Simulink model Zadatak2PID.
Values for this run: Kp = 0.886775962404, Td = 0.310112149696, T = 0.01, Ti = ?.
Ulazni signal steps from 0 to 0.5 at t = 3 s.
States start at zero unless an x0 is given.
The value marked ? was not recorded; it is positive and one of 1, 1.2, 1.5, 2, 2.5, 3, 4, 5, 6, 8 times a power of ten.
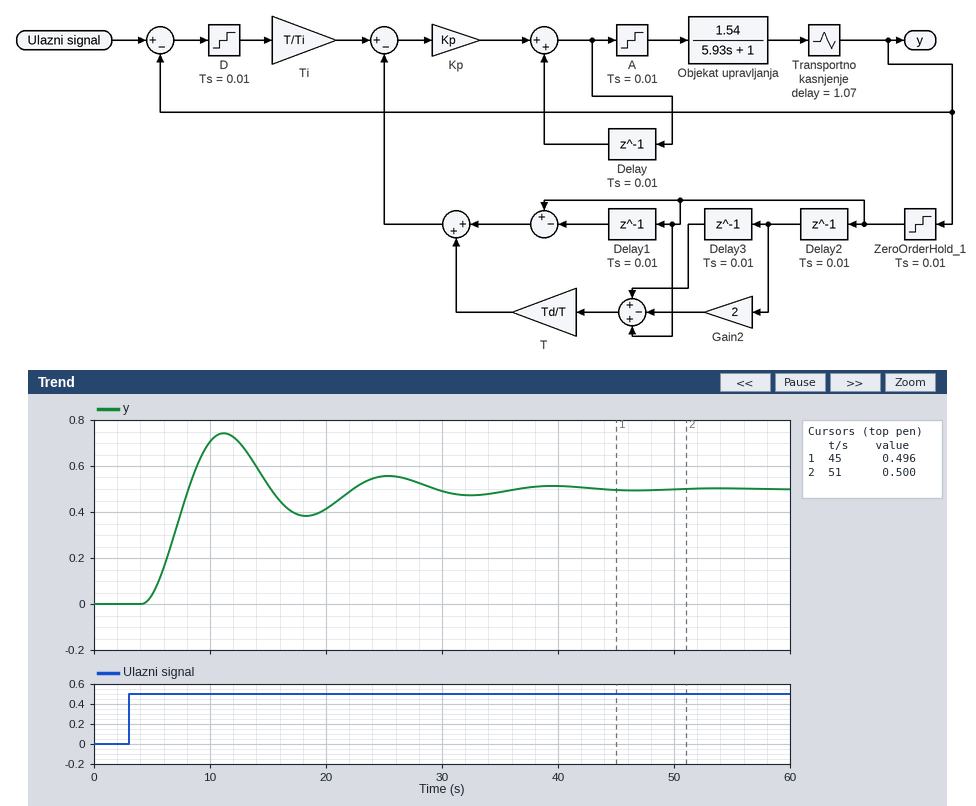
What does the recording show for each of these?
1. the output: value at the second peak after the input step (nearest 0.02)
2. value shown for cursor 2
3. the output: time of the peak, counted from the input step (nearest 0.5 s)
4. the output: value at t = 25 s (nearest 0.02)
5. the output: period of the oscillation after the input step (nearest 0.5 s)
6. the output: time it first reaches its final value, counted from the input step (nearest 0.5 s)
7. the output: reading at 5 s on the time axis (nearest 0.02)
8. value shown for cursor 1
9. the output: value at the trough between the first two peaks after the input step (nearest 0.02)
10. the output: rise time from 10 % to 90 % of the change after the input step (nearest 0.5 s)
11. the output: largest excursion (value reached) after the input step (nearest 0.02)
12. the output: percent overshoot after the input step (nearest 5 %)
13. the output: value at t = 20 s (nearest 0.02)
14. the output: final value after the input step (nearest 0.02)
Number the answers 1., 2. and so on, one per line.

1. 0.56
2. 0.500
3. 8.0 s
4. 0.56
5. 14.0 s
6. 5.0 s
7. 0.04
8. 0.496
9. 0.38
10. 2.5 s
11. 0.74
12. 50 %
13. 0.42
14. 0.50
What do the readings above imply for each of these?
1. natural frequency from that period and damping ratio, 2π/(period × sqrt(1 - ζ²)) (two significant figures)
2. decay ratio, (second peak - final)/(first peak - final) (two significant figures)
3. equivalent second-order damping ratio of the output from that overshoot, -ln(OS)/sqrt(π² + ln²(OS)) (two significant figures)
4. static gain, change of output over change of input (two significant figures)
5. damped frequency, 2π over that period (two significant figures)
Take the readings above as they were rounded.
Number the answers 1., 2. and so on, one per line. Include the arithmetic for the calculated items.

1. 2π / (14 × sqrt(1 - 0.22²)) = 0.46 rad/s
2. (0.56 - 0.5) / (0.74 - 0.5) = 0.25
3. ln(0.5) = -0.693; 0.693 / sqrt(9.870 + 0.480) = 0.22
4. (0.5 - 0) / (0.5 - 0) = 1.0
5. 2π / 14 = 0.45 rad/s
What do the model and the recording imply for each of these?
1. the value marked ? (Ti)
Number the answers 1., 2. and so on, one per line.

1. 1.2
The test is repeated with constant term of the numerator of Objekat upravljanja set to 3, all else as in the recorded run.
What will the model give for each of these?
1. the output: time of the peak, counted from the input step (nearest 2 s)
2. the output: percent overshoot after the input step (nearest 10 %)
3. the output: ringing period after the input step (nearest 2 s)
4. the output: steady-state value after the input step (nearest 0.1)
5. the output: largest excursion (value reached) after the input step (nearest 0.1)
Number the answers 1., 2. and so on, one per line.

1. 6 s
2. 60 %
3. 10 s
4. 0.5
5. 0.8
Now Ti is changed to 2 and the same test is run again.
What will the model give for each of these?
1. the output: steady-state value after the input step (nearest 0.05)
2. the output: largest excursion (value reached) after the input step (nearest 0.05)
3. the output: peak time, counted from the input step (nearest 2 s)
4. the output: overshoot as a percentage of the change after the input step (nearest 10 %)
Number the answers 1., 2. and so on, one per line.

1. 0.50
2. 0.60
3. 10 s
4. 20 %
